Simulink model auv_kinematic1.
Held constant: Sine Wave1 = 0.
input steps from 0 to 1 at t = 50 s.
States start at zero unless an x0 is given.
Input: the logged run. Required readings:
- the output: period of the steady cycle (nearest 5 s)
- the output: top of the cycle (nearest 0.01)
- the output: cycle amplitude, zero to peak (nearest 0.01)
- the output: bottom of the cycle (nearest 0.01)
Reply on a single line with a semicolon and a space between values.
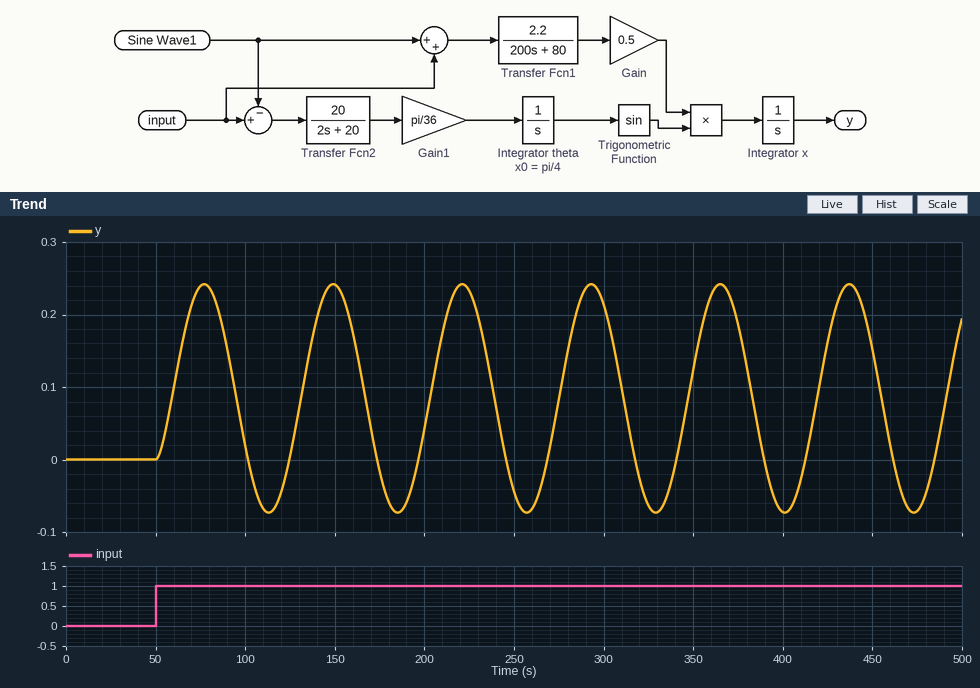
70 s; 0.24; 0.16; -0.07
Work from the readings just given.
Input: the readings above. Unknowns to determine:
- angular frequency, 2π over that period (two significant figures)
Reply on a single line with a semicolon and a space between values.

0.090 rad/s
